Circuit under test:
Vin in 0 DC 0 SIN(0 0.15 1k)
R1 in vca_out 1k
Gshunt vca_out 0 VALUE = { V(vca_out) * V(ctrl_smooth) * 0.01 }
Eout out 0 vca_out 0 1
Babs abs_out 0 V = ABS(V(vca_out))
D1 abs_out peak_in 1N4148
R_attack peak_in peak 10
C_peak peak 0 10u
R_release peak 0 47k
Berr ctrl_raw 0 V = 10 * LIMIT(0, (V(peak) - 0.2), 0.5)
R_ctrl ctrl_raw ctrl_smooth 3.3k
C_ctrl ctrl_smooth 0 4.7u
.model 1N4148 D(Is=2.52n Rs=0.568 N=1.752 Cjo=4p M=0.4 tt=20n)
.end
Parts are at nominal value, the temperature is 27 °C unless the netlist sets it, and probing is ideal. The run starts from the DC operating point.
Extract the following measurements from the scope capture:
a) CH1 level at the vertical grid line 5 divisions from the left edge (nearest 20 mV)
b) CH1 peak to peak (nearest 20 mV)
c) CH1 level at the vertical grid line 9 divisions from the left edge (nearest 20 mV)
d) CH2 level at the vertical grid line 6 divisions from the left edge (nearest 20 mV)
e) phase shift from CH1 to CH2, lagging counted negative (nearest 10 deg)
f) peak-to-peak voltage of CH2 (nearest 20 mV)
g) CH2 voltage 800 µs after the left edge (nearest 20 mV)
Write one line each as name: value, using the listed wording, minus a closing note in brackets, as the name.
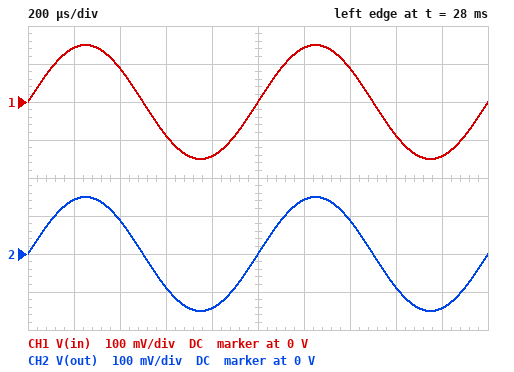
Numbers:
CH1 level at the vertical grid line 5 divisions from the left edge: 0 V
CH1 peak to peak: 300 mV
CH1 level at the vertical grid line 9 divisions from the left edge: -140 mV
CH2 level at the vertical grid line 6 divisions from the left edge: 140 mV
phase shift from CH1 to CH2, lagging counted negative: 0 deg
peak-to-peak voltage of CH2: 300 mV
CH2 voltage 800 µs after the left edge: -140 mV
